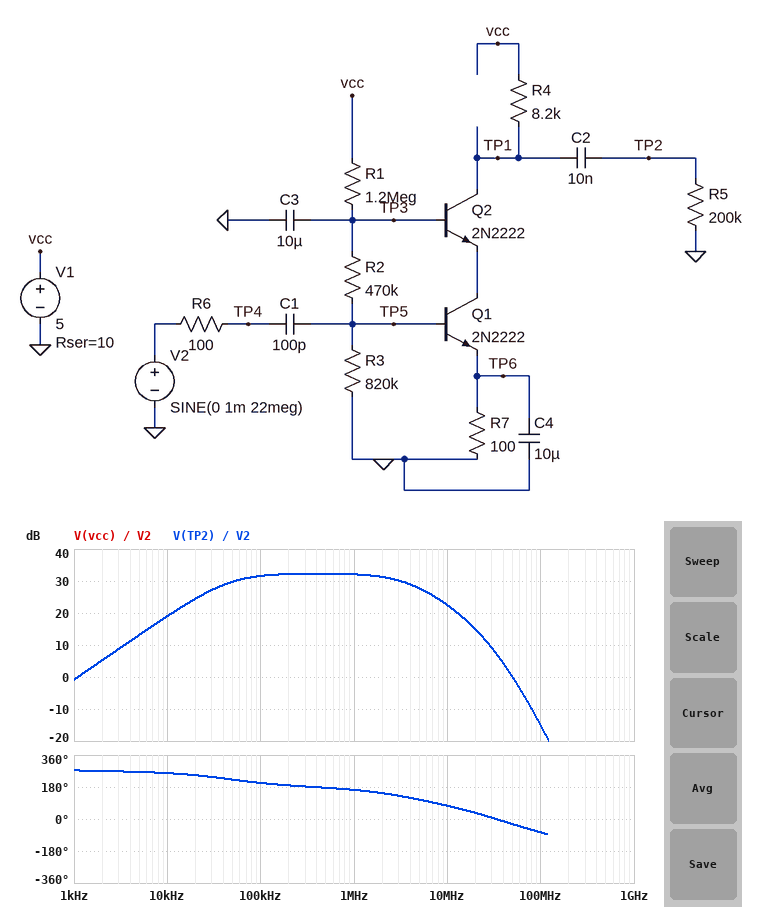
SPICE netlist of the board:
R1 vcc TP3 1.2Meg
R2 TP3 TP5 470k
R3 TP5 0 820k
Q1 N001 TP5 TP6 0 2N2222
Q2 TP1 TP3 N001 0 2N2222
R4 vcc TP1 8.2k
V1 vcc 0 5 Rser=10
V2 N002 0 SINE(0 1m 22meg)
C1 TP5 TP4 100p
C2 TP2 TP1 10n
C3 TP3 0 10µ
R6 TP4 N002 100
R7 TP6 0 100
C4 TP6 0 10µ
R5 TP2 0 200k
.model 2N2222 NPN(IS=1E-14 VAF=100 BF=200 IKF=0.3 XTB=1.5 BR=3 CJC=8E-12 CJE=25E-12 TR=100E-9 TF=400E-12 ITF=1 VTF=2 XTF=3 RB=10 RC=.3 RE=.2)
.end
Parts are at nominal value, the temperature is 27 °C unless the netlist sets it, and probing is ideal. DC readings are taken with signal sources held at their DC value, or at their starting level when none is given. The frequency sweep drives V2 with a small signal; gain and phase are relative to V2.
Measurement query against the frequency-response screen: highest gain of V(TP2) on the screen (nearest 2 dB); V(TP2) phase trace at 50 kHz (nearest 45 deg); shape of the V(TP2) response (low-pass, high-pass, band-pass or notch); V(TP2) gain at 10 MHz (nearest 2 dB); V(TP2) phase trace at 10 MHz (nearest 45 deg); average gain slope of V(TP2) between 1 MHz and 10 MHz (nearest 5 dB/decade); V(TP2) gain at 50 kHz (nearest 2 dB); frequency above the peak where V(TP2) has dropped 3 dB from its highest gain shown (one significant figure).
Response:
32 dB
225 deg
band-pass
22 dB
90 deg
-10 dB/decade
30 dB
4 MHz
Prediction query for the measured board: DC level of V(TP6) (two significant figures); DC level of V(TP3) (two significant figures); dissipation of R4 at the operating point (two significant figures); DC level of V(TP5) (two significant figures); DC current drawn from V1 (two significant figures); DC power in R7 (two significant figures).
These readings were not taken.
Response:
22 mV
1.5 V
380 µW
640 mV
220 µA
4.7 µW
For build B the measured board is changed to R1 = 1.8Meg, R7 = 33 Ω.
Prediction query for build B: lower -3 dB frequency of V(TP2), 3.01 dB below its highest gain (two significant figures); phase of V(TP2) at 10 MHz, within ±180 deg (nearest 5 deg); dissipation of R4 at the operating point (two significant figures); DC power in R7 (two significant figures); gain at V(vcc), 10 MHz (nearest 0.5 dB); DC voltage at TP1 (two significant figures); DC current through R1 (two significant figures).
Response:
30 kHz
65 deg
150 µW
610 nW
-39.5 dB
3.9 V
2.1 µA
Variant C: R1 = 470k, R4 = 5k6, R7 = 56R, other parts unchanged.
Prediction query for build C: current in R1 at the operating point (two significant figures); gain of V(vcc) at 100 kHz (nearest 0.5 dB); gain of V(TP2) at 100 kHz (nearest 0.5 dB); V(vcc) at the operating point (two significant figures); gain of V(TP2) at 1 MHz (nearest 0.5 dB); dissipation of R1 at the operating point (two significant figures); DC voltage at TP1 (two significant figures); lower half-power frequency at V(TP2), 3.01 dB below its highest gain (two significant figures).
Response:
5.9 µA
-21.5 dB
33.5 dB
5.0 V
36.0 dB
16 µW
2.2 V
95 kHz
